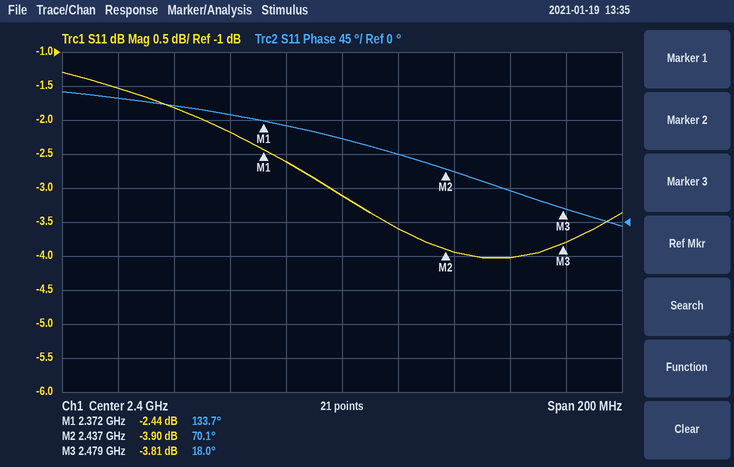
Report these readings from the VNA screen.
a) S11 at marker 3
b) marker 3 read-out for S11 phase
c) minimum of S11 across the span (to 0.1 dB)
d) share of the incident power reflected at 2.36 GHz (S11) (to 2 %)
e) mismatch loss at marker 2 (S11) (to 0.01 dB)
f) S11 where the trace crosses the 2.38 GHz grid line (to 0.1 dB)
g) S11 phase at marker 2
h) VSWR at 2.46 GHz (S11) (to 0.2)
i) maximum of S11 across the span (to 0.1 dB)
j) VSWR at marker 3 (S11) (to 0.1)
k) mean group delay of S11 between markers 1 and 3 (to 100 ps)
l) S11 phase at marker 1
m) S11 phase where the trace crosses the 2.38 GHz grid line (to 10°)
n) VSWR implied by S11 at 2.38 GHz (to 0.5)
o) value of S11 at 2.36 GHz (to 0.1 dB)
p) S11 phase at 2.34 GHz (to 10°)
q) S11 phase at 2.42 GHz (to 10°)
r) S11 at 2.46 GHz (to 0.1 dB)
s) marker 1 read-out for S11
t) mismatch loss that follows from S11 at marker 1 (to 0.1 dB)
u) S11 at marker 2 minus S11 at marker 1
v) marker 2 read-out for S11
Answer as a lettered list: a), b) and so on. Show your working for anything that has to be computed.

a) -3.81 dB
b) 18.0°
c) -4.0 dB
d) 10^(-2.2/10) ≈ 60 %
e) −10 log10(1 − 10^(-3.9/10)) ≈ 2.27 dB
f) -2.6 dB
g) 70.1°
h) |Γ| = 10^(-4/20) = 0.6310; VSWR = (1 + 0.6310)/(1 − 0.6310) ≈ 4.4
i) -1.3 dB
j) (1 + 0.6449)/(1 − 0.6449) ≈ 4.6
k) −(18° − (133.7°))/(360° × 107 MHz) ≈ 3.0 ns
l) 133.7°
m) 130°
n) |Γ| = 10^(-2.6/20) = 0.7413; VSWR = (1 + 0.7413)/(1 − 0.7413) ≈ 6.73, so 6.5 to the nearest 0.5
o) -2.2 dB
p) 150°
q) 90°
r) -4.0 dB
s) -2.44 dB
t) −10 log10(1 − 10^(-2.44/10)) ≈ 3.7 dB
u) -3.9 − (-2.44) = -1.46 dB
v) -3.90 dB
